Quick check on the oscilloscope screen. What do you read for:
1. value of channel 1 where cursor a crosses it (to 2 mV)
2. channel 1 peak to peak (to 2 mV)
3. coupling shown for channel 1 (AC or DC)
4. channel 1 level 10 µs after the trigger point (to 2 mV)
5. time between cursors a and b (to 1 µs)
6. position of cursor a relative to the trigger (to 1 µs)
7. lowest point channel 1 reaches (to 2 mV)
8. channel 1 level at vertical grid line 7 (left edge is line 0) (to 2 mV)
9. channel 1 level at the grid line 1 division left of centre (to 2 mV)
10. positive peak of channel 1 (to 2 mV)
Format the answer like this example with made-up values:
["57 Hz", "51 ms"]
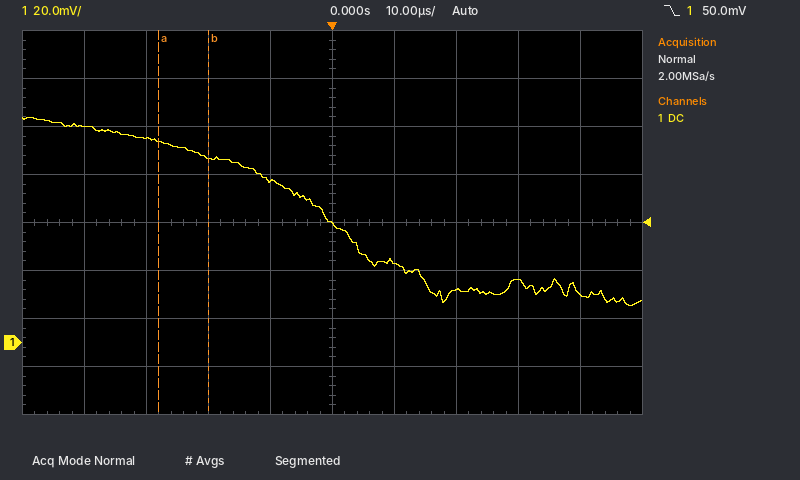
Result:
["84 mV", "78 mV", "DC", "34 mV", "8 µs", "-28 µs", "16 mV", "22 mV", "68 mV", "94 mV"]
